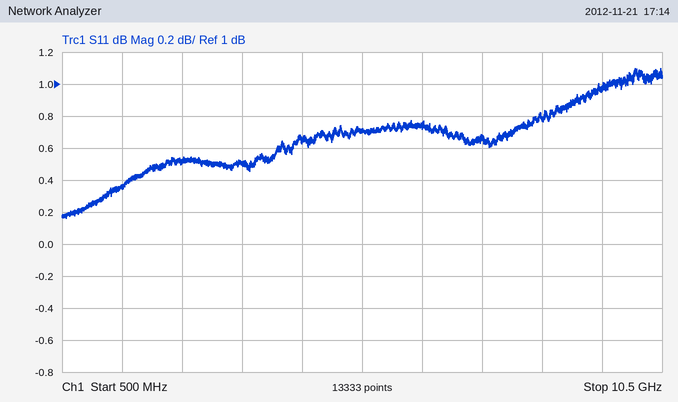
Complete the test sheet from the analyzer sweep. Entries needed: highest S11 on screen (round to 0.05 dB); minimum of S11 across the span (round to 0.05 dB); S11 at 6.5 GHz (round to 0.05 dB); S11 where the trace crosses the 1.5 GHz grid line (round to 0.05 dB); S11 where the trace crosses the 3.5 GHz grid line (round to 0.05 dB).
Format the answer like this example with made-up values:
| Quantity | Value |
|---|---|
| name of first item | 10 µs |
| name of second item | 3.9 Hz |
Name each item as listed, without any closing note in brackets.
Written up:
| Quantity | Value |
|---|---|
| highest S11 on screen | 1.10 dB |
| minimum of S11 across the span | 0.15 dB |
| S11 at 6.5 GHz | 0.75 dB |
| S11 where the trace crosses the 1.5 GHz grid line | 0.35 dB |
| S11 where the trace crosses the 3.5 GHz grid line | 0.50 dB |
